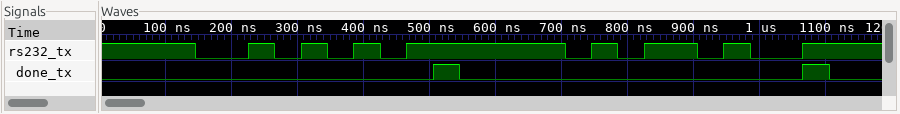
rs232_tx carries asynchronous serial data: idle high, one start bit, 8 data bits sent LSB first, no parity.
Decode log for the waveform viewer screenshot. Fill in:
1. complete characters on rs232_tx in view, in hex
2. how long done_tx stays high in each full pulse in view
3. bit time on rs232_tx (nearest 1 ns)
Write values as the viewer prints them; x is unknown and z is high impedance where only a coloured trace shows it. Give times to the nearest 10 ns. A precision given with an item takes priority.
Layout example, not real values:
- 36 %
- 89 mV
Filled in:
- AA, 2D
- 40 ns, 40 ns
- 40 ns
